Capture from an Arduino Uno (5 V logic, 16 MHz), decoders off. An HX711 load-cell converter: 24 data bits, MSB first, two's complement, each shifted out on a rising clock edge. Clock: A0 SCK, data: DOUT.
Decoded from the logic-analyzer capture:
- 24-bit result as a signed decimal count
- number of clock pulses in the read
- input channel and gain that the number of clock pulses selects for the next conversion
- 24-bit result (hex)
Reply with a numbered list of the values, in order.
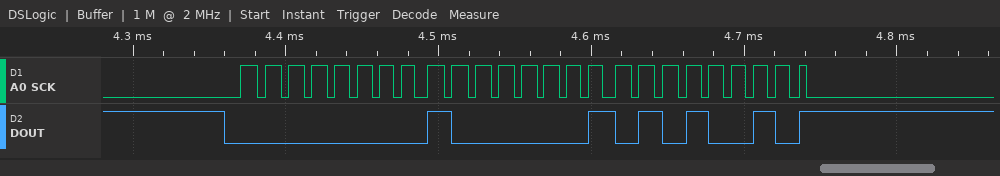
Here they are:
1. 33106
2. 25
3. channel A, gain 128
4. 0x008152
